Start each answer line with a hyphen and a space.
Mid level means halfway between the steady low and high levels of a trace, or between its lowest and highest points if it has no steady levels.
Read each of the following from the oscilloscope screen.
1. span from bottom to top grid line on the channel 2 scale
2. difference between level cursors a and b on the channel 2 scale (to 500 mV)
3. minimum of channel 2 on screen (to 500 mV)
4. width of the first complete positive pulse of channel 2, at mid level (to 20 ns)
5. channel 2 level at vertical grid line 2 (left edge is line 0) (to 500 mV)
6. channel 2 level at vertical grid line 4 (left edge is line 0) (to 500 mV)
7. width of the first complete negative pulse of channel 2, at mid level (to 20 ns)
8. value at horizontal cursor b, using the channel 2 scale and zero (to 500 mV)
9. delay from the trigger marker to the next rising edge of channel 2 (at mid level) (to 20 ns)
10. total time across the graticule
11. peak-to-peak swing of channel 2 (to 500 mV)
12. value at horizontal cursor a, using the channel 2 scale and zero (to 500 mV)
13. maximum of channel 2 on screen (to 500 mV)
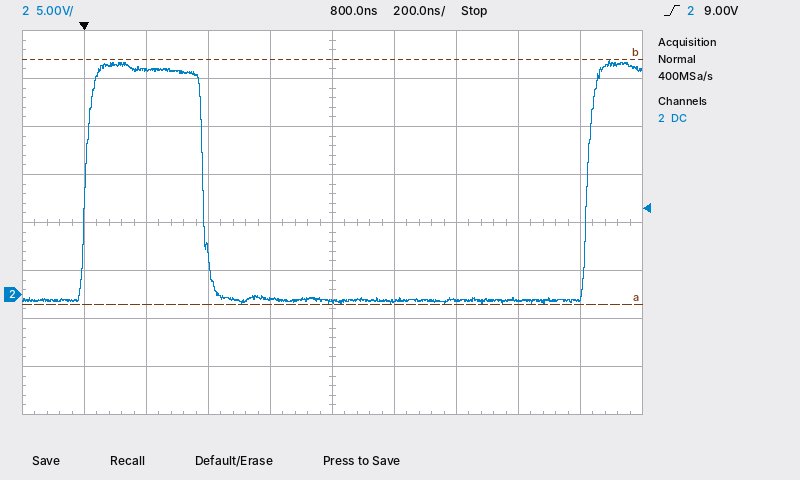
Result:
- 40 V
- 25.5 V
- -1.0 V
- 380 ns
- 23.5 V
- -500 mV
- 1.24 µs
- 24.5 V
- 1.62 µs
- 2 µs
- 25.5 V
- -1.0 V
- 24.5 V
